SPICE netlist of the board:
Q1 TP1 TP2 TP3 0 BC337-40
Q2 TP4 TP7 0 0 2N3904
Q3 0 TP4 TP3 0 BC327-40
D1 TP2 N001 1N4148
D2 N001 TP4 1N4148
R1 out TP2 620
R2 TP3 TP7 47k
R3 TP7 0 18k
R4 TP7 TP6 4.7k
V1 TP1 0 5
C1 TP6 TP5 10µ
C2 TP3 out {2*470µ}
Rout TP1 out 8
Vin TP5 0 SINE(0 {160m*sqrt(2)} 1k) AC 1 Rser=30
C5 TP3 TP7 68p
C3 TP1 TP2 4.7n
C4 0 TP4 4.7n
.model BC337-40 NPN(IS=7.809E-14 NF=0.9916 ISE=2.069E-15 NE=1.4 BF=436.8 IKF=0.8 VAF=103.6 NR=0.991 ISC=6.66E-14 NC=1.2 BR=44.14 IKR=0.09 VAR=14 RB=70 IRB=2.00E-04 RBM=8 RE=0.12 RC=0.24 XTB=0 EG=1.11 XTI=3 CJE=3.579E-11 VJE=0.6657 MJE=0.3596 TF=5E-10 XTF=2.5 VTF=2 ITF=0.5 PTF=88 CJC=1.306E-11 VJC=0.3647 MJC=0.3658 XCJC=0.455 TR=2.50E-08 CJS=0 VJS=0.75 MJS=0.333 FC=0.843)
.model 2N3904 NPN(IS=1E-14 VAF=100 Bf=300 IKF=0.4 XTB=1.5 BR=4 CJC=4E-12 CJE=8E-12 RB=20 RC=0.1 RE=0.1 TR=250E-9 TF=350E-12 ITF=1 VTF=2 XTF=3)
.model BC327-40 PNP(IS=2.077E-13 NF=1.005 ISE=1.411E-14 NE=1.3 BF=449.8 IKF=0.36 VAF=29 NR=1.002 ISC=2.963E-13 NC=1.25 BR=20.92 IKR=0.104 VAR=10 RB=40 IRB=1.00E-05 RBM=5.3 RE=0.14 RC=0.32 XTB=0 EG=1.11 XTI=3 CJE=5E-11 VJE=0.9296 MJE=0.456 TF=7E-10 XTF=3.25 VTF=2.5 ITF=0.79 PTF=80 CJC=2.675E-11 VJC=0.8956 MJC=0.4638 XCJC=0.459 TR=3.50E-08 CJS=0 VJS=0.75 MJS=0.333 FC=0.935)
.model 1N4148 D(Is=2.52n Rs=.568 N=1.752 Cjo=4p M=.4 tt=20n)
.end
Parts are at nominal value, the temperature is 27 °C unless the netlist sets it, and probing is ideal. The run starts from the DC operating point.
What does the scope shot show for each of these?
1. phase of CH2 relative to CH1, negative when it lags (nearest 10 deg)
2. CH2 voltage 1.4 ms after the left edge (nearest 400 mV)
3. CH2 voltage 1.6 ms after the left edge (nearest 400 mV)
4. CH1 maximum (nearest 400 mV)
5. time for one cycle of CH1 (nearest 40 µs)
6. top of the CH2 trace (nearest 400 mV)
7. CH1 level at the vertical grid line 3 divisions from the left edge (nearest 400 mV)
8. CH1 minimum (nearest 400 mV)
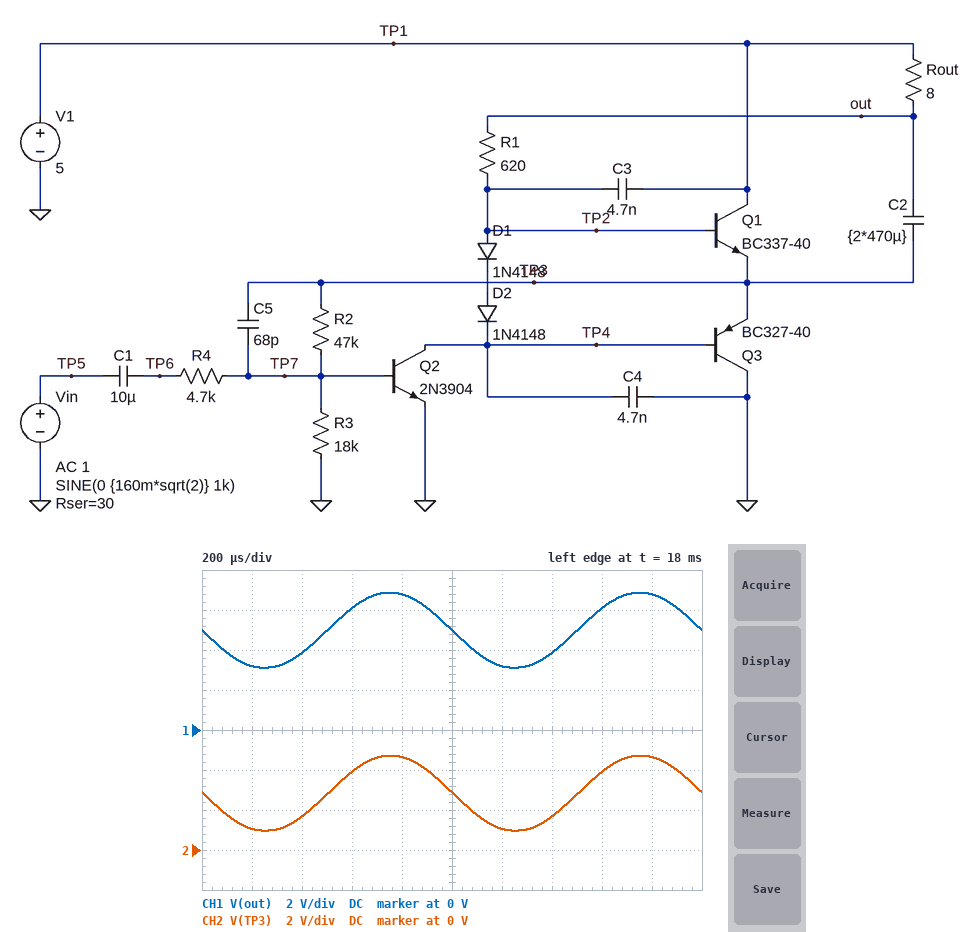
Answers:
0 deg
1.6 V
4.0 V
6.8 V
1.00 ms
4.8 V
6.0 V
3.2 V
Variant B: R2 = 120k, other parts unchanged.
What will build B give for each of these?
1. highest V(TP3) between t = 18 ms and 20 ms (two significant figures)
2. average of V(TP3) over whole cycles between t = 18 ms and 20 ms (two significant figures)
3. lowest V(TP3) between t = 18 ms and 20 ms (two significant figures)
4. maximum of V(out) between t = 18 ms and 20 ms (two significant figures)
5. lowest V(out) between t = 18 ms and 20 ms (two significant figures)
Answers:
4.8 V
4.1 V
2.4 V
5.7 V
3.3 V
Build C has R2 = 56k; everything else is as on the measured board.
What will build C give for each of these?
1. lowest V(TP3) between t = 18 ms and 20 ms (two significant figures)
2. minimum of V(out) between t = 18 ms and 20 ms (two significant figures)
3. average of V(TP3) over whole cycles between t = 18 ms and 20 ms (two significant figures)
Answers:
1.0 V
2.9 V
3.1 V
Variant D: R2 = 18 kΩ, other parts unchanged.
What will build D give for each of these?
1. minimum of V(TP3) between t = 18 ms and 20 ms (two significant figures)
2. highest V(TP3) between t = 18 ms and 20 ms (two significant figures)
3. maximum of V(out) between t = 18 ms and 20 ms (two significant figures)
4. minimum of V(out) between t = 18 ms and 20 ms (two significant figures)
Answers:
880 mV
2.5 V
5.8 V
4.2 V
